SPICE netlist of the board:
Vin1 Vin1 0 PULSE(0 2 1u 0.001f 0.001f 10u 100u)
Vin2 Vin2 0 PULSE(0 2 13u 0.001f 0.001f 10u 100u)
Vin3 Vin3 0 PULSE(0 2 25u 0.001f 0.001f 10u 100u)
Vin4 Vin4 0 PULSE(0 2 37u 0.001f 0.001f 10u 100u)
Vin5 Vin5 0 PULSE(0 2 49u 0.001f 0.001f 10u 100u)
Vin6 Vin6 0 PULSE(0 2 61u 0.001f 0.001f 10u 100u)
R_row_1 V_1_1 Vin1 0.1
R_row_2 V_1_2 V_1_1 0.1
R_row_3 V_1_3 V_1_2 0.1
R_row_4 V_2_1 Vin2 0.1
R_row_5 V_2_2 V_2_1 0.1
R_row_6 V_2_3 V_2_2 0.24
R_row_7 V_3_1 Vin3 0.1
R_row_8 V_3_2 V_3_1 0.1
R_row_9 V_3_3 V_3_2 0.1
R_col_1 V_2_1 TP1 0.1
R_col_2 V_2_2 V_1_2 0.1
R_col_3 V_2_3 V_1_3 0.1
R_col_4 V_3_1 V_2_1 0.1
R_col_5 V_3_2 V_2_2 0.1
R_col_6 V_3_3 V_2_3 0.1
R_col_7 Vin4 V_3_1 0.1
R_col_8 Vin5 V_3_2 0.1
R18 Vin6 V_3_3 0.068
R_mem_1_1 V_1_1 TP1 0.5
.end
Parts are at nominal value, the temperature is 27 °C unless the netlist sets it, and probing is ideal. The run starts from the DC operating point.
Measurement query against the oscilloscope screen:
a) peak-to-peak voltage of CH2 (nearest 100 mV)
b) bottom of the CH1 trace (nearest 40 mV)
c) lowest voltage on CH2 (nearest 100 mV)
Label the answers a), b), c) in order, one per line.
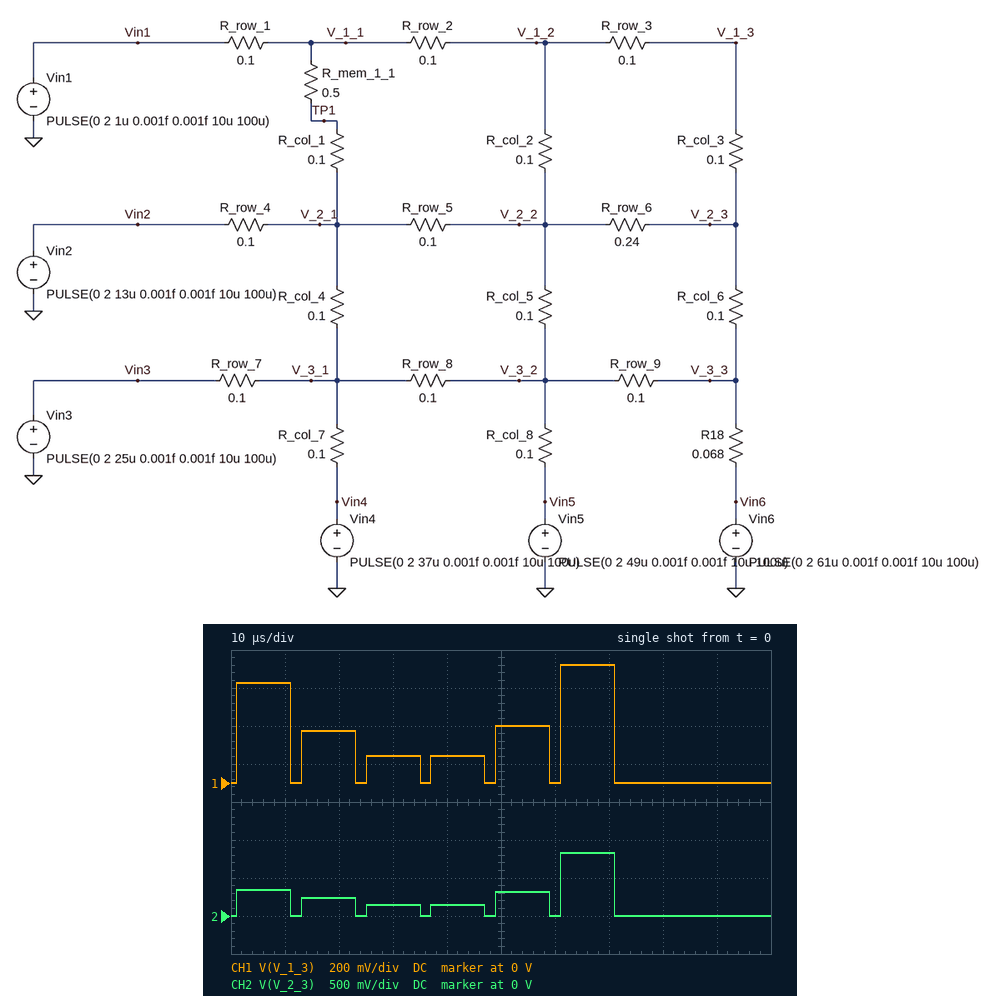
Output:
a) 800 mV
b) 0 V
c) 0 V
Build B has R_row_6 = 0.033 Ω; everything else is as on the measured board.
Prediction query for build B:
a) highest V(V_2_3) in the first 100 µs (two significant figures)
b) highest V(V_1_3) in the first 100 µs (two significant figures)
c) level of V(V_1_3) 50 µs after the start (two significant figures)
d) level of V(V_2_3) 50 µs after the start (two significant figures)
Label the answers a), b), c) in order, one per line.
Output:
a) 640 mV
b) 530 mV
c) 320 mV
d) 350 mV
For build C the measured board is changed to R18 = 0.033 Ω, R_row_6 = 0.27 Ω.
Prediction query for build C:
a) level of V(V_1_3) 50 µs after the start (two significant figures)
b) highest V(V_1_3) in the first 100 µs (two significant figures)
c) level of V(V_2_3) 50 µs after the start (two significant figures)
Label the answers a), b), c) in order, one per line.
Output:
a) 240 mV
b) 780 mV
c) 230 mV
